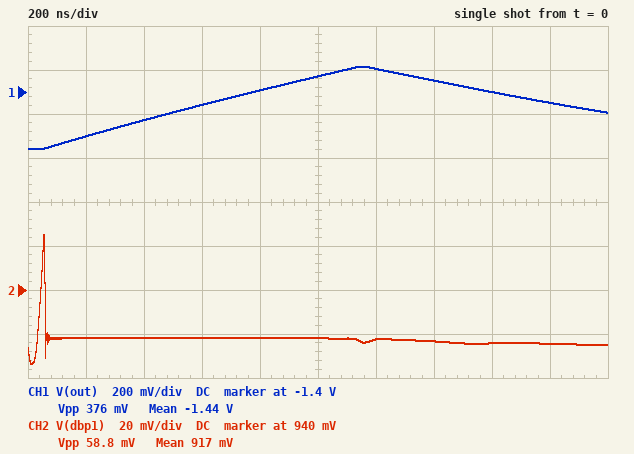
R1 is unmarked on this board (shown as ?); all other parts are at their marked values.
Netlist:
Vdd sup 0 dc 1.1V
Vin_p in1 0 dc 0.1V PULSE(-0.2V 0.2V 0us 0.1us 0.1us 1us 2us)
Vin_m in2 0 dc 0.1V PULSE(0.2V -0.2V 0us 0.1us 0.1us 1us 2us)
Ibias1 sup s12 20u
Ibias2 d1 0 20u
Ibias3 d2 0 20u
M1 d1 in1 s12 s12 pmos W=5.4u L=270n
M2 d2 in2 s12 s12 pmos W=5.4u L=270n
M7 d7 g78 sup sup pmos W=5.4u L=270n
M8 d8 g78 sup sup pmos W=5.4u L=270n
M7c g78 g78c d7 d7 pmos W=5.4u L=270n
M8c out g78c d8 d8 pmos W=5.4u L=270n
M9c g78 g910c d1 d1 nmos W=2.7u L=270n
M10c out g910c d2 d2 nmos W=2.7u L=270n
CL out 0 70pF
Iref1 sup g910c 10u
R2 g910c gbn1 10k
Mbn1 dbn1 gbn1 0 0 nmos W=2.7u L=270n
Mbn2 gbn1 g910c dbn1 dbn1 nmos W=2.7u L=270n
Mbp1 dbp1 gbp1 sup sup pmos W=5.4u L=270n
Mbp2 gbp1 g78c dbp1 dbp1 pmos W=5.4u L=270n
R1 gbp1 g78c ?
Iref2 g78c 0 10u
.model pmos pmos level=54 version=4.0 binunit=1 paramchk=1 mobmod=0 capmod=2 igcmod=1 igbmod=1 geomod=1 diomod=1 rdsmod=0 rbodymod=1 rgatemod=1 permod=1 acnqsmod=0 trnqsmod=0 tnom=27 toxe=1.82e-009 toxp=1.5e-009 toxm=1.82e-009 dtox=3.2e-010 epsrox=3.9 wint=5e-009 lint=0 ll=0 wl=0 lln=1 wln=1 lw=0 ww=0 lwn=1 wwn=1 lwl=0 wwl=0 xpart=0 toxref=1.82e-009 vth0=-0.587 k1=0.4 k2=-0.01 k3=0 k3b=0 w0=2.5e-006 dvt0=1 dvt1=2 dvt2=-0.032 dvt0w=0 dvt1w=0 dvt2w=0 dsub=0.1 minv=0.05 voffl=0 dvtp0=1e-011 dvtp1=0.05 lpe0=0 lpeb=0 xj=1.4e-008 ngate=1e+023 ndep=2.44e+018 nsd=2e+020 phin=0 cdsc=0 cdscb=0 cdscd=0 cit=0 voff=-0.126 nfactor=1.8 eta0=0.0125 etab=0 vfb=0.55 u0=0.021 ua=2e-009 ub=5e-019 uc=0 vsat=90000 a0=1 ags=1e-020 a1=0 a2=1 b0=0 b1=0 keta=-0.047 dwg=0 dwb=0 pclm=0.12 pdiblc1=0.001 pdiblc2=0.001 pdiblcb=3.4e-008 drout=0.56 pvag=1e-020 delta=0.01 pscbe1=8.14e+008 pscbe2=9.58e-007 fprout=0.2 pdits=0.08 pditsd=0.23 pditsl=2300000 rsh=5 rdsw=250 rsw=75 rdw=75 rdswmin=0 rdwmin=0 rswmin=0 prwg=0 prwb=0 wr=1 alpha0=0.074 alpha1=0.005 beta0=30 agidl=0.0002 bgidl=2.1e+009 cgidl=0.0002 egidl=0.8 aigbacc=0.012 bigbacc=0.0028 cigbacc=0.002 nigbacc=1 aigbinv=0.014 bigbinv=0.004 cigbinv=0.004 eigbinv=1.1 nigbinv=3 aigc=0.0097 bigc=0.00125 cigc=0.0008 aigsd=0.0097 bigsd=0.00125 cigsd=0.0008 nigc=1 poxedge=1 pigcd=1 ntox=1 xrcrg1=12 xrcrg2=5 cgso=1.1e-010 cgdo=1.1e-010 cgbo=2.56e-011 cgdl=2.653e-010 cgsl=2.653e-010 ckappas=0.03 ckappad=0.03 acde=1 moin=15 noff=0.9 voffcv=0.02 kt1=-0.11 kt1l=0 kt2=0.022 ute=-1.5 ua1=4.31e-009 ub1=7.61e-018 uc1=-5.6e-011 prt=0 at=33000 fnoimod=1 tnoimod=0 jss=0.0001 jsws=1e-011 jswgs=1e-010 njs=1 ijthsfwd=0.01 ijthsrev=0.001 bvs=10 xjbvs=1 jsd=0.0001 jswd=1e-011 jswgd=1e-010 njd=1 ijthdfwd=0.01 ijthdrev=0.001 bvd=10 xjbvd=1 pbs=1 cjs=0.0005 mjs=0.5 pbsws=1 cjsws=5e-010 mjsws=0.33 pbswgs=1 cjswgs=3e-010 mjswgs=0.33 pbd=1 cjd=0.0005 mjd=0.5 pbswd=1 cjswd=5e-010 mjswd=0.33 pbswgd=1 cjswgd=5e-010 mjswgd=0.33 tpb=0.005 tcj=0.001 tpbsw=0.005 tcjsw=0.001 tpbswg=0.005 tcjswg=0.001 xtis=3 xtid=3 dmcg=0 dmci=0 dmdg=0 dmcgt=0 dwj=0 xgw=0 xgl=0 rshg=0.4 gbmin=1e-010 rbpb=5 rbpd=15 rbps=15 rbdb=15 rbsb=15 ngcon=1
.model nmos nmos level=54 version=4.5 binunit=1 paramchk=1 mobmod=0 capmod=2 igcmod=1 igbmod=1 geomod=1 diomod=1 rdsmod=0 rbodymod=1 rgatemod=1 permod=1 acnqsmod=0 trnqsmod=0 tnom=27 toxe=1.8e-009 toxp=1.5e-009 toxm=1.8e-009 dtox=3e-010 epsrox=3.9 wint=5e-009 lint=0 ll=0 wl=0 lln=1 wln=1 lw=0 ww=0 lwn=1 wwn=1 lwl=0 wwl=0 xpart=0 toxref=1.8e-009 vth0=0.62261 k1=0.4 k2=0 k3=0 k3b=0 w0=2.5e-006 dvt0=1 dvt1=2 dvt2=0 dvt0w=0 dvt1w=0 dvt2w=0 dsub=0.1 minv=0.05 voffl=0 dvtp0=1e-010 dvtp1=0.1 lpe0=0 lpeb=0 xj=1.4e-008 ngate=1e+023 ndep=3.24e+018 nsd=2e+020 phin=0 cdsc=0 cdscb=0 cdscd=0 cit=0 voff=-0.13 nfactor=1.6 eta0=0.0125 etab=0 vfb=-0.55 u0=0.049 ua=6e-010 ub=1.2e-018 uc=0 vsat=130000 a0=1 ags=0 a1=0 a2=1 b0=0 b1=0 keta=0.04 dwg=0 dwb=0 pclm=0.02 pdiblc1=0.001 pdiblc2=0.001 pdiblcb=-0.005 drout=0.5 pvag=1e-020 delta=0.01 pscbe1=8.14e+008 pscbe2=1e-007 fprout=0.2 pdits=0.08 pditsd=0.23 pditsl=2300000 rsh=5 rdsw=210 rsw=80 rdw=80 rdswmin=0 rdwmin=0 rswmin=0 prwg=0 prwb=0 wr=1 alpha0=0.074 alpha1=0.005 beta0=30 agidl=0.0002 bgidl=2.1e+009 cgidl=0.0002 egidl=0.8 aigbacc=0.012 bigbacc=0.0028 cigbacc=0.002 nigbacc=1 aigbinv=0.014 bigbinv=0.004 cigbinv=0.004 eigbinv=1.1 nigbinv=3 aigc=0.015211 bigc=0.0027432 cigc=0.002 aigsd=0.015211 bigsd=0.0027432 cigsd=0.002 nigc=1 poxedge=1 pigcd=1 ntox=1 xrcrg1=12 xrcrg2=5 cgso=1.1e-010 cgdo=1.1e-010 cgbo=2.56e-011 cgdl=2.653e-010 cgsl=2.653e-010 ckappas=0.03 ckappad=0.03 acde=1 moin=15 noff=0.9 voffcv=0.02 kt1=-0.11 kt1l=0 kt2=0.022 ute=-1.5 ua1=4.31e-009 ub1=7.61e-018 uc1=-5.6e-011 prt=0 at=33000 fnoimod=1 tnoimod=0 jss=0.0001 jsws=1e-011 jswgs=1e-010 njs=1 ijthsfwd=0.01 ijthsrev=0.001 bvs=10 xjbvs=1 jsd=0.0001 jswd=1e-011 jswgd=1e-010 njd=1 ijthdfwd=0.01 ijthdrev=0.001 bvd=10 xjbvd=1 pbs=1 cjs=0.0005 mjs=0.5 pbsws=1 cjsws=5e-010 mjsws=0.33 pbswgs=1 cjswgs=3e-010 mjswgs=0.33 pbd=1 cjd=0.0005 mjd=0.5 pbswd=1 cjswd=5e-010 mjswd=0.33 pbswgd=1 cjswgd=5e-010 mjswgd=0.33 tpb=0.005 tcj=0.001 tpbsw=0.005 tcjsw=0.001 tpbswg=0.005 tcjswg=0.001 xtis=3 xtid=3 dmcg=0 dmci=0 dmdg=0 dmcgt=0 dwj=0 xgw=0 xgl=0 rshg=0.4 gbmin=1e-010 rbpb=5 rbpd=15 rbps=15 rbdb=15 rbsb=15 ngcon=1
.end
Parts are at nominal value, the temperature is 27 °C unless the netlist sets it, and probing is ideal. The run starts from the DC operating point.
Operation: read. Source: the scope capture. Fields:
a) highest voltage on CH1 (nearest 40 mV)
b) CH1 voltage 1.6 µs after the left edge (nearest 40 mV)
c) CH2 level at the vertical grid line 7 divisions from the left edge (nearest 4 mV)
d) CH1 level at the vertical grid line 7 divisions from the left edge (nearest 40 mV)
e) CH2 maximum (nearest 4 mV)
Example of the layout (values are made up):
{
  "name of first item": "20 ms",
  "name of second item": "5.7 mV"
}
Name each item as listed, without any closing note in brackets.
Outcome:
{
  "highest voltage on CH1": "-1.28 V",
  "CH1 voltage 1.6 µs after the left edge": "-1.40 V",
  "CH2 level at the vertical grid line 7 divisions from the left edge": "916 mV",
  "CH1 level at the vertical grid line 7 divisions from the left edge": "-1.36 V",
  "CH2 maximum": "964 mV"
}
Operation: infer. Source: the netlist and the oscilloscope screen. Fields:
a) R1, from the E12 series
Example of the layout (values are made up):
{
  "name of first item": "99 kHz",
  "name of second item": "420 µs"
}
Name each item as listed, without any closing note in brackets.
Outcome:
{
  "R1, from the E12 series": "18 kΩ"
}
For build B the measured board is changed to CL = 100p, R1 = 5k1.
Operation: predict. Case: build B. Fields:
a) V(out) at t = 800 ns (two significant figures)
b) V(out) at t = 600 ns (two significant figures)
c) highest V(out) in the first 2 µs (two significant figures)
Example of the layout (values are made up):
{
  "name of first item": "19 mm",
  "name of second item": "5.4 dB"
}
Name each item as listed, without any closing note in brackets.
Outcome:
{
  "V(out) at t = 800 ns": "-1.2 V",
  "V(out) at t = 600 ns": "-1.3 V",
  "highest V(out) in the first 2 µs": "-1.1 V"
}
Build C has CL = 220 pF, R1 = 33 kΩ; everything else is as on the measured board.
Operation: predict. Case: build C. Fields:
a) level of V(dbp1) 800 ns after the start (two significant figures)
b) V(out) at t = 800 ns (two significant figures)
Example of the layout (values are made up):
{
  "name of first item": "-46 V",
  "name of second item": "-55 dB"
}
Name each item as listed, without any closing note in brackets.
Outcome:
{
  "level of V(dbp1) 800 ns after the start": "770 mV",
  "V(out) at t = 800 ns": "-1.6 V"
}
